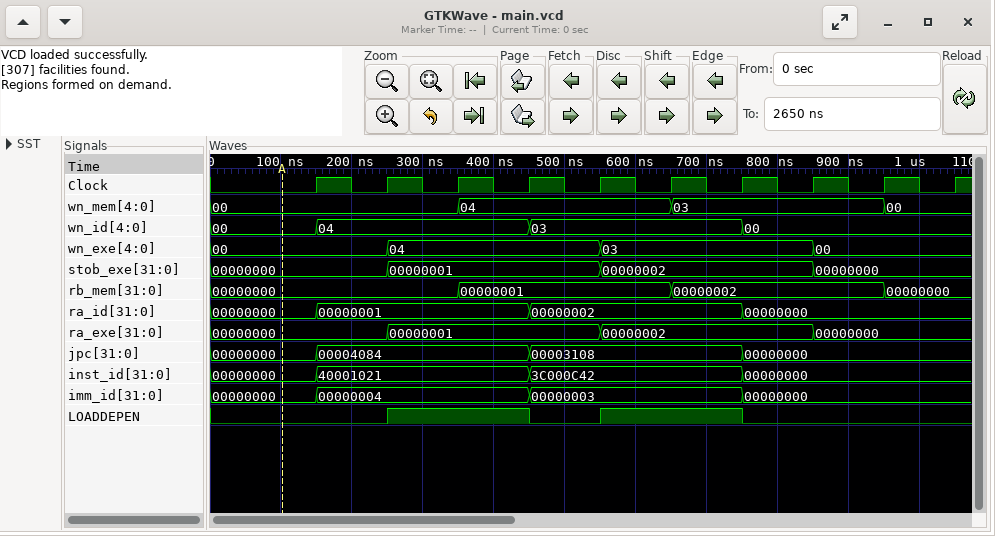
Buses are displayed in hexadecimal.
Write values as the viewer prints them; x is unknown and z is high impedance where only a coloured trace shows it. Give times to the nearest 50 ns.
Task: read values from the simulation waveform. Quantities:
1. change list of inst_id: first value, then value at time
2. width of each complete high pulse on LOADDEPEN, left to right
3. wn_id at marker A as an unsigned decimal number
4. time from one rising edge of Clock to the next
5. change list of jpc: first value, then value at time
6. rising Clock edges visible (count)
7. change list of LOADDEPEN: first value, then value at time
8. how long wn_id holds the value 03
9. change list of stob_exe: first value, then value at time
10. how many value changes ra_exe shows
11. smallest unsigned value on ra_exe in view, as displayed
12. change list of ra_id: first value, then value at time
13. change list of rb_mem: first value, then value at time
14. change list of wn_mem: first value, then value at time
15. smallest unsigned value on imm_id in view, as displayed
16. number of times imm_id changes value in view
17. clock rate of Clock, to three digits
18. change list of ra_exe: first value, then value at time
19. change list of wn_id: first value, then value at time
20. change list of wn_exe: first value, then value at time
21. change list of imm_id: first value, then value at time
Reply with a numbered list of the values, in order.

1. 00000000, 40001021 at 150 ns, 3C000C42 at 450 ns, 00000000 at 750 ns
2. 200 ns, 200 ns
3. 0
4. 100 ns
5. 00000000, 00004084 at 150 ns, 00003108 at 450 ns, 00000000 at 750 ns
6. 10
7. 0, 1 at 250 ns, 0 at 450 ns, 1 at 550 ns, 0 at 750 ns
8. 300 ns
9. 00000000, 00000001 at 250 ns, 00000002 at 550 ns, 00000000 at 850 ns
10. 3
11. 00000000
12. 00000000, 00000001 at 150 ns, 00000002 at 450 ns, 00000000 at 750 ns
13. 00000000, 00000001 at 350 ns, 00000002 at 650 ns, 00000000 at 950 ns
14. 00, 04 at 350 ns, 03 at 650 ns, 00 at 950 ns
15. 00000000
16. 3
17. 10.0 MHz
18. 00000000, 00000001 at 250 ns, 00000002 at 550 ns, 00000000 at 850 ns
19. 00, 04 at 150 ns, 03 at 450 ns, 00 at 750 ns
20. 00, 04 at 250 ns, 03 at 550 ns, 00 at 850 ns
21. 00000000, 00000004 at 150 ns, 00000003 at 450 ns, 00000000 at 750 ns
